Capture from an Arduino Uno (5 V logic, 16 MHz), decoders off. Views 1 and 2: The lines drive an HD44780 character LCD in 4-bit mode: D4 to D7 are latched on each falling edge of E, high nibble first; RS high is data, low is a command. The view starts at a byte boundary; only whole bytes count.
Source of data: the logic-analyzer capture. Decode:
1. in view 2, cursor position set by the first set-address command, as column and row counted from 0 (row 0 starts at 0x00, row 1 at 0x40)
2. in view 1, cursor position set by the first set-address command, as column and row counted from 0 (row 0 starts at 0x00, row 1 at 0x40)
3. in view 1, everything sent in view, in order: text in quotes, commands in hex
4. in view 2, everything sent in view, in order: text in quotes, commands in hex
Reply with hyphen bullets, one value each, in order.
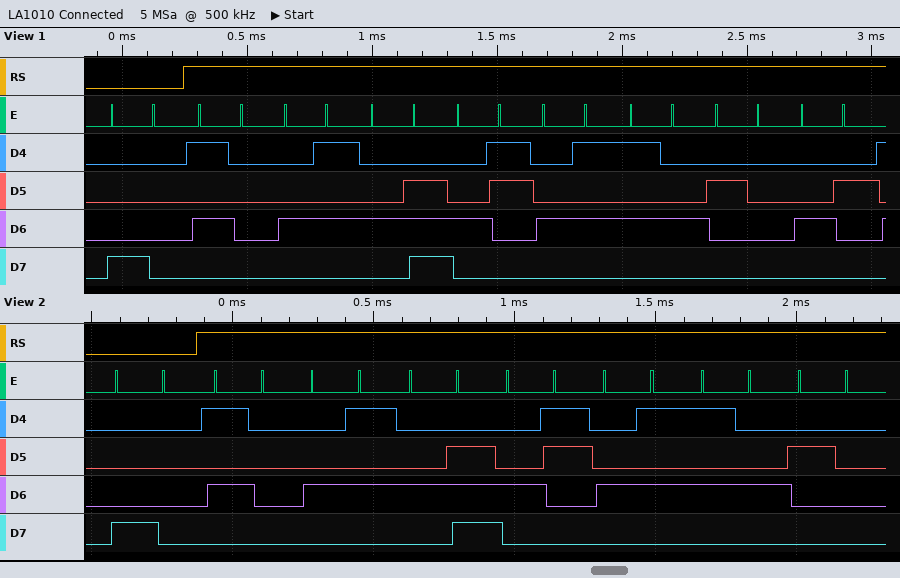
- column 0, row 0
- column 0, row 0
- 0x80 "PENCET B"
- 0x80 "PENCET "
